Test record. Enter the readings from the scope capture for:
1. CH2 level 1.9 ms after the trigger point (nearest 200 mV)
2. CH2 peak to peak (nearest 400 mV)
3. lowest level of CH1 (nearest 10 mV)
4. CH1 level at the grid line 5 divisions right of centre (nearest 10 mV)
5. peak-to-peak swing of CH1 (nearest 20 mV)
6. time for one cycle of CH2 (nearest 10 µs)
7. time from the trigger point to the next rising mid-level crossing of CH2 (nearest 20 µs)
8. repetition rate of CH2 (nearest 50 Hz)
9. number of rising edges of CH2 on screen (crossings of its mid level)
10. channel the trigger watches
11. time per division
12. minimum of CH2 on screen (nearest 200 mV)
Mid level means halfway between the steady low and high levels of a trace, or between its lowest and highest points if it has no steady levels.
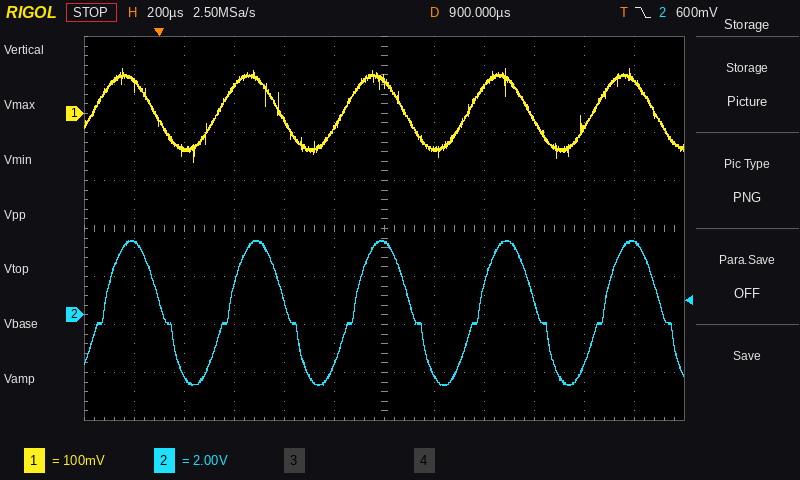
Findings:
3.0 V
6.0 V
-100 mV
70 mV
200 mV
500 µs
280 µs
2.00 kHz
5
CH2
200 µs
-3.0 V
